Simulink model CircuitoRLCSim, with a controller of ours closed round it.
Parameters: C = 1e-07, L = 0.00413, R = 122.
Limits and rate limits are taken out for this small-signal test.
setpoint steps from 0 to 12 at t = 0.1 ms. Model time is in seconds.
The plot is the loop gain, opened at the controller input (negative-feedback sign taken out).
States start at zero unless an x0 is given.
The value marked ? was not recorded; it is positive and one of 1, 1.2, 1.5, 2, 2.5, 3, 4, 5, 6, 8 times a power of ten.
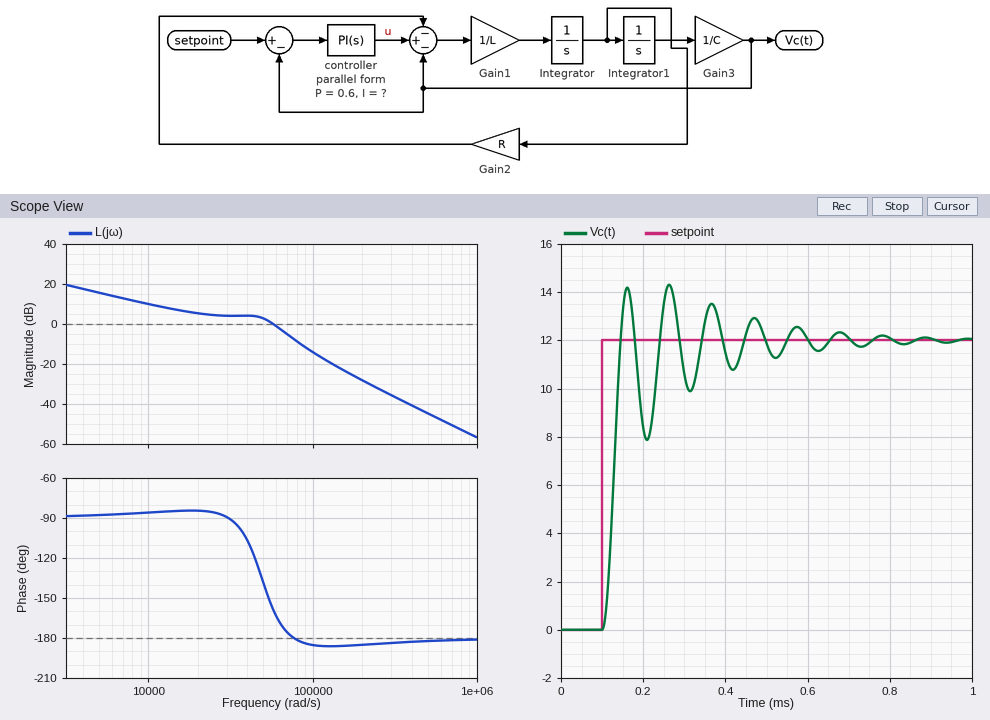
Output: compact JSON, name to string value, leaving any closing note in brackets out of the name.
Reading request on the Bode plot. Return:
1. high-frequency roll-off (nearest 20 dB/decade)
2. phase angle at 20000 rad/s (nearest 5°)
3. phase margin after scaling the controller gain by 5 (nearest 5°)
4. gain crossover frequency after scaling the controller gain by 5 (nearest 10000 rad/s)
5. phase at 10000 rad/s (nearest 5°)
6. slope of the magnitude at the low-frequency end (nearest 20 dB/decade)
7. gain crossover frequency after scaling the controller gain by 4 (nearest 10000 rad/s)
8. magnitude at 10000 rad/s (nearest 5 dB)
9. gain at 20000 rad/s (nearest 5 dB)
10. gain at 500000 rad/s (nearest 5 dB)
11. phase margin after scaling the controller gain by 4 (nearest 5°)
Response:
{"high-frequency roll-off": "-40 dB/decade", "phase angle at 20000 rad/s": "-85°", "phase margin after scaling the controller gain by 5": "-5°", "gain crossover frequency after scaling the controller gain by 5": "100000 rad/s", "phase at 10000 rad/s": "-85°", "slope of the magnitude at the low-frequency end": "-20 dB/decade", "gain crossover frequency after scaling the controller gain by 4": "90000 rad/s", "magnitude at 10000 rad/s": "10 dB", "gain at 20000 rad/s": "5 dB", "gain at 500000 rad/s": "-45 dB", "phase margin after scaling the controller gain by 4": "-5°"}
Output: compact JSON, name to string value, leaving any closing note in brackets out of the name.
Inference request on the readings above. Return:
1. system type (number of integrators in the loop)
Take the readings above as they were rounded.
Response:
{"system type": "1"}
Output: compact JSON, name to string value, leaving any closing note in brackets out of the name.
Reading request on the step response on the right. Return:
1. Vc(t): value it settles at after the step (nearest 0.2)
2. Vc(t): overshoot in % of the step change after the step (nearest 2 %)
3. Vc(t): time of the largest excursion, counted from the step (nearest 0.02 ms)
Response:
{"Vc(t): value it settles at after the step": "12.0", "Vc(t): overshoot in % of the step change after the step": "20 %", "Vc(t): time of the largest excursion, counted from the step": "0.16 ms"}
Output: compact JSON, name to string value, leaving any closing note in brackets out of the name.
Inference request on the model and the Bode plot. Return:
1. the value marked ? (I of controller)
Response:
{"the value marked ?": "30000"}
